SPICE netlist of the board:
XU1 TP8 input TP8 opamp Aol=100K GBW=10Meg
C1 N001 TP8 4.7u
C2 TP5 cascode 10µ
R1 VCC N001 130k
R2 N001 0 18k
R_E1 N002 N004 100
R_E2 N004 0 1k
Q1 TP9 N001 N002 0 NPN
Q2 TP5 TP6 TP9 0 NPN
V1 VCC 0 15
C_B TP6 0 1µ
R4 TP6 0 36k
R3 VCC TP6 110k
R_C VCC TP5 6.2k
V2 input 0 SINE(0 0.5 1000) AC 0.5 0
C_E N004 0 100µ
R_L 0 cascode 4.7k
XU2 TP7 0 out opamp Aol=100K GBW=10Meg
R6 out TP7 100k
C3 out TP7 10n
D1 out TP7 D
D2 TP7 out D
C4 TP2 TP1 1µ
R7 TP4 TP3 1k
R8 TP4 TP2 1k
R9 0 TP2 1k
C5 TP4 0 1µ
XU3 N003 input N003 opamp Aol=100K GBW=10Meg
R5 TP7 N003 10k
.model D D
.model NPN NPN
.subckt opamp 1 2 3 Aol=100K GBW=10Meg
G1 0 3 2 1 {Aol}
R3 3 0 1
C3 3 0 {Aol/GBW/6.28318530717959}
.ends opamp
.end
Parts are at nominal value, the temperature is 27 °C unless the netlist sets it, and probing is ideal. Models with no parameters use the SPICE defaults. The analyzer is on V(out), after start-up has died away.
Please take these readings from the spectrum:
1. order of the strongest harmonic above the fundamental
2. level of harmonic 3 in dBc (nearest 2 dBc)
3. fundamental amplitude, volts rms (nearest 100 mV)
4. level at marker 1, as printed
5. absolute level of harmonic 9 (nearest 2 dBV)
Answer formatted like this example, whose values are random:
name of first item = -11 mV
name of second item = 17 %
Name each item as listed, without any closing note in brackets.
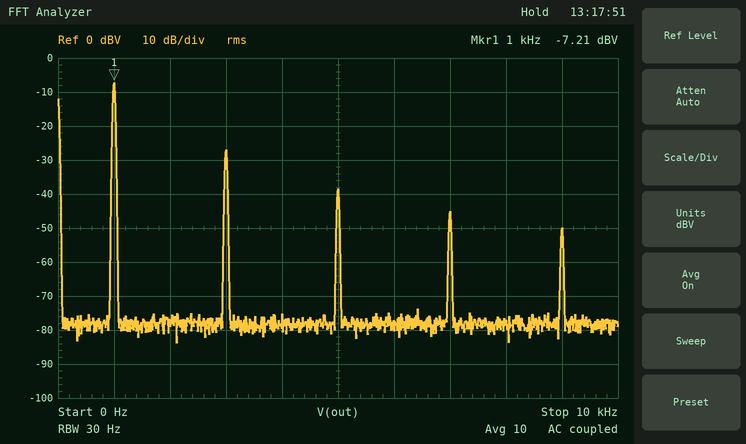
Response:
order of the strongest harmonic above the fundamental = 3
level of harmonic 3 in dBc = -20 dBc
fundamental amplitude, volts rms = 400 mV
level at marker 1, as printed = -7.21 dBV
absolute level of harmonic 9 = -50 dBV
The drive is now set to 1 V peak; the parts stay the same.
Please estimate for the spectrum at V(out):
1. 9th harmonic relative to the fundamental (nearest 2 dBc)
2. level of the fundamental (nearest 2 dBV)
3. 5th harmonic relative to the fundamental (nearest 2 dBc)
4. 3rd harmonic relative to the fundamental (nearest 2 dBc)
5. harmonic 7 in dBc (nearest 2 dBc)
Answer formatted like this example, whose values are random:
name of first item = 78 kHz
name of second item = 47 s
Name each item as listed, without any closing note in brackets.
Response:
9th harmonic relative to the fundamental = -36 dBc
level of the fundamental = -6 dBV
5th harmonic relative to the fundamental = -26 dBc
3rd harmonic relative to the fundamental = -14 dBc
harmonic 7 in dBc = -32 dBc
